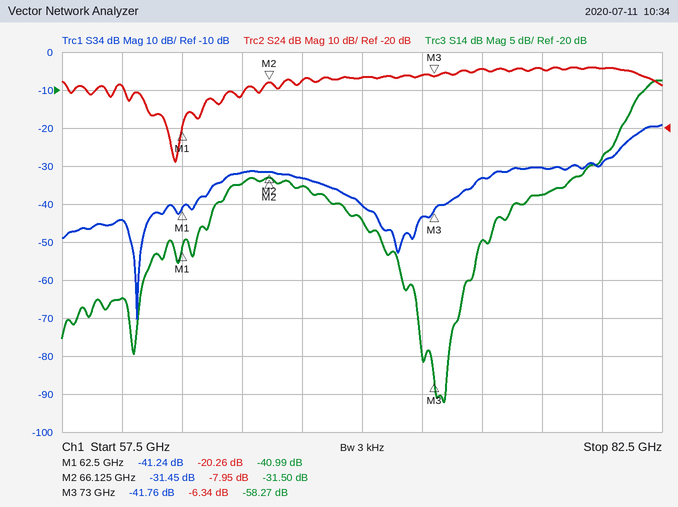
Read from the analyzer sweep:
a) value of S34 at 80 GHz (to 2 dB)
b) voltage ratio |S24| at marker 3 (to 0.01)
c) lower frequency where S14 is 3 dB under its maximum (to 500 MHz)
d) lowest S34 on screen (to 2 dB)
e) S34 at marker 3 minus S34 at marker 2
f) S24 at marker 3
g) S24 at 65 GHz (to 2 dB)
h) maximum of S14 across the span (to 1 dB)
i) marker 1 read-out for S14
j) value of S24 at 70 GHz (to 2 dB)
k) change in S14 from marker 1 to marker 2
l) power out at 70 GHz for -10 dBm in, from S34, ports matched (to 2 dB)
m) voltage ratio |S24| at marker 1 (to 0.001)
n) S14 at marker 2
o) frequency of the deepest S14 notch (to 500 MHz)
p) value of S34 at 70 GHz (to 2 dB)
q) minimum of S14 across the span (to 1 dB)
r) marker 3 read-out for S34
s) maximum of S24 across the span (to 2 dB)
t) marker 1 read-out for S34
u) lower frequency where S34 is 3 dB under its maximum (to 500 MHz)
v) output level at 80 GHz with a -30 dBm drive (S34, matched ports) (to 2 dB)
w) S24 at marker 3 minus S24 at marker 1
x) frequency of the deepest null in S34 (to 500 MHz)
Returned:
-30 dB
0.48
81.5 GHz
-70 dB
-10.31 dB
-6.34 dB
-12 dB
-19 dB
-40.99 dB
-6 dB
9.49 dB
-50 dBm
0.097
-31.50 dB
73.5 GHz
-40 dB
-61 dB
-41.76 dB
-4 dB
-41.24 dB
81.5 GHz
-60 dBm
13.92 dB
60.5 GHz
